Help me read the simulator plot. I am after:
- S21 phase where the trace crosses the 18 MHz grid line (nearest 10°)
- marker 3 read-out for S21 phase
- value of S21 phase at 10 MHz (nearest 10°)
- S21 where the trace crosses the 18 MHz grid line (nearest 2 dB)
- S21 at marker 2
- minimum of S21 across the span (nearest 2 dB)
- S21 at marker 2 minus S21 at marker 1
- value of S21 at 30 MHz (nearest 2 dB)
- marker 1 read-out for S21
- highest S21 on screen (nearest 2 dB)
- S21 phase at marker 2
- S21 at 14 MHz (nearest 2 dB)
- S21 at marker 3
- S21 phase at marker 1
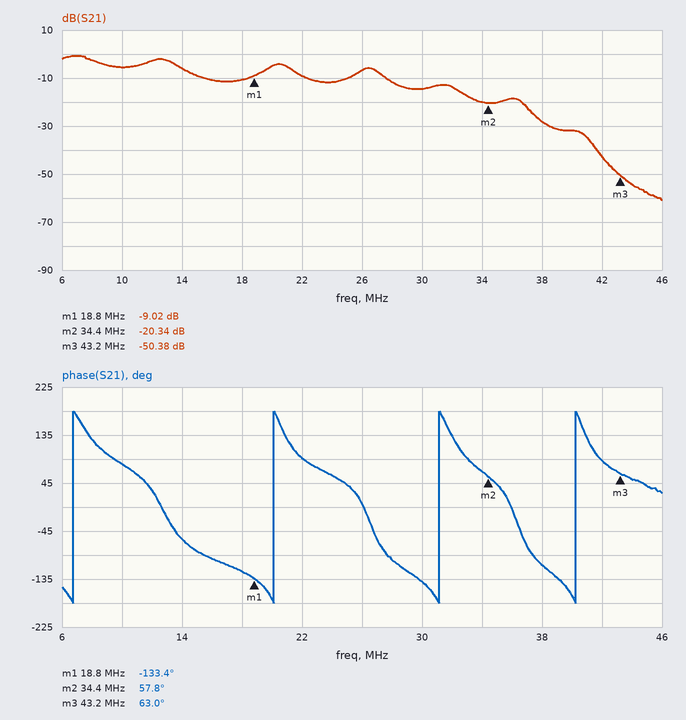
-120°
63.0°
80°
-10 dB
-20.34 dB
-60 dB
-11.32 dB
-14 dB
-9.02 dB
0 dB
57.8°
-6 dB
-50.38 dB
-133.4°
